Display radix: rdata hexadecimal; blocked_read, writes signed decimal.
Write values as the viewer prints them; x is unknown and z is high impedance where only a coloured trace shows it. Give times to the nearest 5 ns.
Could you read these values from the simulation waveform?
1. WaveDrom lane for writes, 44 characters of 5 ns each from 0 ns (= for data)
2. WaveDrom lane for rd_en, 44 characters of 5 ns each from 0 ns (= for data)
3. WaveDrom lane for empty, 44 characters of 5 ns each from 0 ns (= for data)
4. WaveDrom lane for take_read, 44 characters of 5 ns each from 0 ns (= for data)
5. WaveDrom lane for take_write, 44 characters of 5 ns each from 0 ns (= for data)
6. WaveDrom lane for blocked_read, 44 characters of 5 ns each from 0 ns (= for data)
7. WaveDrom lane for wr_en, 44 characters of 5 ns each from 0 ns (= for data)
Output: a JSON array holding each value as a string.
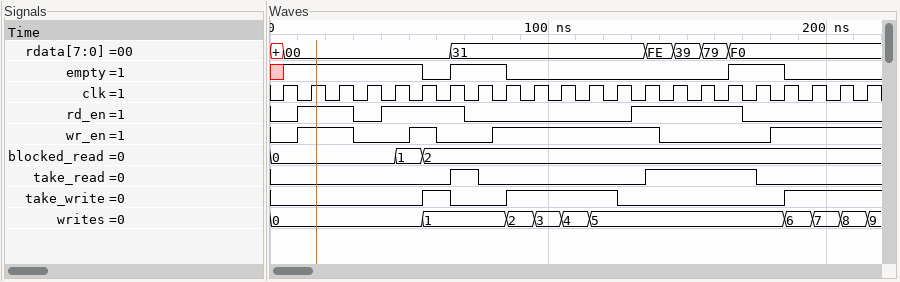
["{name: 'writes', wave: '=..........=.....=.=.=.=.............=.=.=.=', data: '0 1 2 3 4 5 6 7 8 9'}", "{name: 'rd_en', wave: '0.1...0.1.....0...........1.......0.........'}", "{name: 'empty', wave: 'x1.........0.1...0...............1...0......'}", "{name: 'take_read', wave: '0............1.0...........1.......0........'}", "{name: 'take_write', wave: '0..........1.0...1.......0...........1......'}", "{name: 'blocked_read', wave: '=........=.=................................', data: '0 1 2'}", "{name: 'wr_en', wave: '0.1...0...1.0...1...........0.......1.......'}"]
